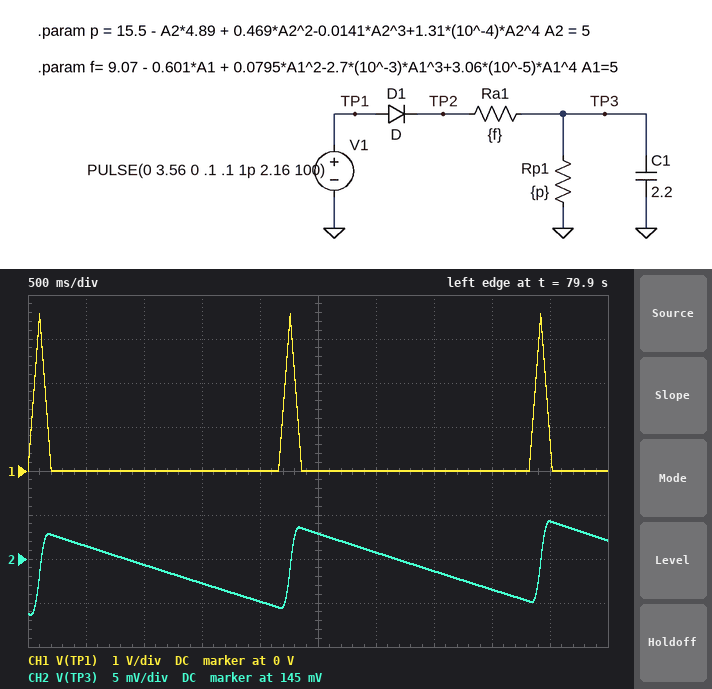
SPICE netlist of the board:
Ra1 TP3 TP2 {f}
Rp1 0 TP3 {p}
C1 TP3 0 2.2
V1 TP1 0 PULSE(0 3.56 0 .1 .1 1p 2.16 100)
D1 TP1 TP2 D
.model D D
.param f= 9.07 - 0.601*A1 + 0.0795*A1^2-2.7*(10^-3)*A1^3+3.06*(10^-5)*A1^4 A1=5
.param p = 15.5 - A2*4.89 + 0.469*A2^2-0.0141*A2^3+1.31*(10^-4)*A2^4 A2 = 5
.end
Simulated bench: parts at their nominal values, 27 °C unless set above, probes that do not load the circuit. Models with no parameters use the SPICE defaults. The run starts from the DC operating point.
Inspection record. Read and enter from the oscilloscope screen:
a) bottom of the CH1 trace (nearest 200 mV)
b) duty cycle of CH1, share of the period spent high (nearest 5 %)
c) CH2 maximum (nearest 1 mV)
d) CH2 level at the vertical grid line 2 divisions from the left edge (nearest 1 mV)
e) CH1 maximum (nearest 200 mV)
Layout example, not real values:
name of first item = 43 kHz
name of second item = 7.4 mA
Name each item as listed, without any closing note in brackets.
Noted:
bottom of the CH1 trace = 0 V
duty cycle of CH1, share of the period spent high = 5 %
CH2 maximum = 149 mV
CH2 level at the vertical grid line 2 divisions from the left edge = 144 mV
CH1 maximum = 3.6 V
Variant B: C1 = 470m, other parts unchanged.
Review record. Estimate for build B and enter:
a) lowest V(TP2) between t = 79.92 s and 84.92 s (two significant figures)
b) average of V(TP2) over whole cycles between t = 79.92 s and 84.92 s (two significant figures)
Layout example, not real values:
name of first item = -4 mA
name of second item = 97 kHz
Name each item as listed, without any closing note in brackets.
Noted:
lowest V(TP2) between t = 79.92 s and 84.92 s = 130 mV
average of V(TP2) over whole cycles between t = 79.92 s and 84.92 s = 240 mV
